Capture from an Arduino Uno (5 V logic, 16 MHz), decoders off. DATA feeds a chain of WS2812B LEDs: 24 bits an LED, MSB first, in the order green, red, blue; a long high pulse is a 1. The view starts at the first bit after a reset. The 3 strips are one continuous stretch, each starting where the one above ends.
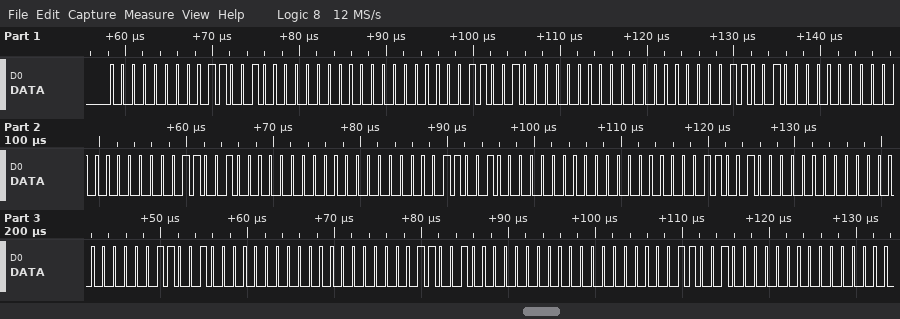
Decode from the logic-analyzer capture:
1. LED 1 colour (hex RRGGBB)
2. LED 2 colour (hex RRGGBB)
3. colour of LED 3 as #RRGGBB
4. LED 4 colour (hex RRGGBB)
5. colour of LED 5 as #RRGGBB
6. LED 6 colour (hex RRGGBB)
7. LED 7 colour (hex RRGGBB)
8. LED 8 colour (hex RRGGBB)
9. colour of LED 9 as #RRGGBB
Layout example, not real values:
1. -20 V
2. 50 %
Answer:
1. #640000
2. #640000
3. #640000
4. #640000
5. #640000
6. #640000
7. #640000
8. #640000
9. #640000
